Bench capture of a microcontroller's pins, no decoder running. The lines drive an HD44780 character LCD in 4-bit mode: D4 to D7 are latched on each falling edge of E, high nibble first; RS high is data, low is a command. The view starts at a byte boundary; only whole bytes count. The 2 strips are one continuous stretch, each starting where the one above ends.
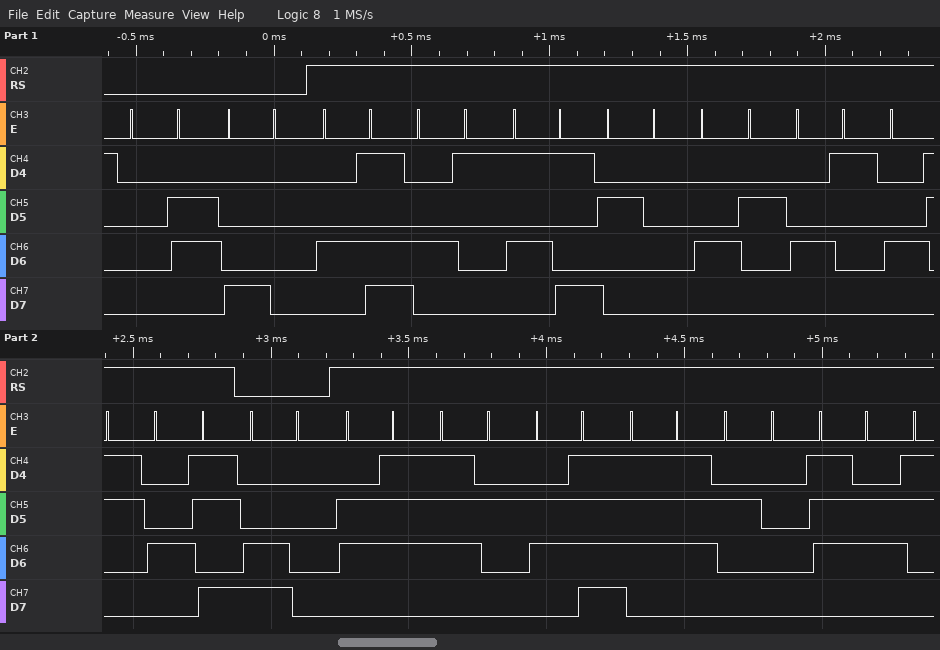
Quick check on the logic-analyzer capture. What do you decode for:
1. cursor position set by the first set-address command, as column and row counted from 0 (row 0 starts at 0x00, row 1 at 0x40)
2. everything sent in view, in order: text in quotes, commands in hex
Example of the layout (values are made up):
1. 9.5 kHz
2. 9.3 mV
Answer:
1. column 0, row 0
2. 0x06 0x80 "MAY BACK" 0xC0 "grow v"
